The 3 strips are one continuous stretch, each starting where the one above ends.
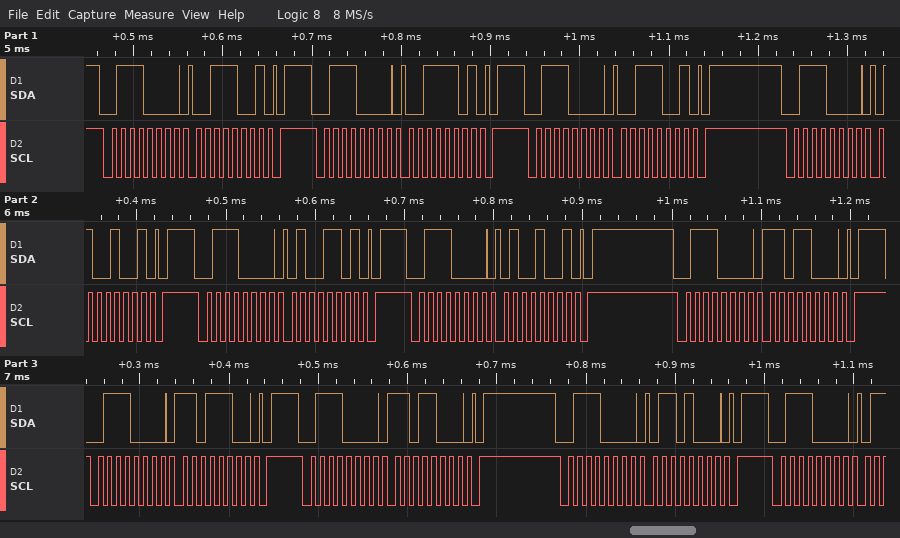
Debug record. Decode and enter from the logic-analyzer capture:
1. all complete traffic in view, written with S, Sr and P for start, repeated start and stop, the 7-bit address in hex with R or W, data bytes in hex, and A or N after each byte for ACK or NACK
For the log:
S 38W A 39 A P S 38W A 3D A P S 38W A 39 A P S 38W A 49 A P S 38W A 4D A P S 38W A 49 A P S 38W A D8 A P S 38W A DC A P S 38W A D8 A P S 38W A 68 A P S 38W A
